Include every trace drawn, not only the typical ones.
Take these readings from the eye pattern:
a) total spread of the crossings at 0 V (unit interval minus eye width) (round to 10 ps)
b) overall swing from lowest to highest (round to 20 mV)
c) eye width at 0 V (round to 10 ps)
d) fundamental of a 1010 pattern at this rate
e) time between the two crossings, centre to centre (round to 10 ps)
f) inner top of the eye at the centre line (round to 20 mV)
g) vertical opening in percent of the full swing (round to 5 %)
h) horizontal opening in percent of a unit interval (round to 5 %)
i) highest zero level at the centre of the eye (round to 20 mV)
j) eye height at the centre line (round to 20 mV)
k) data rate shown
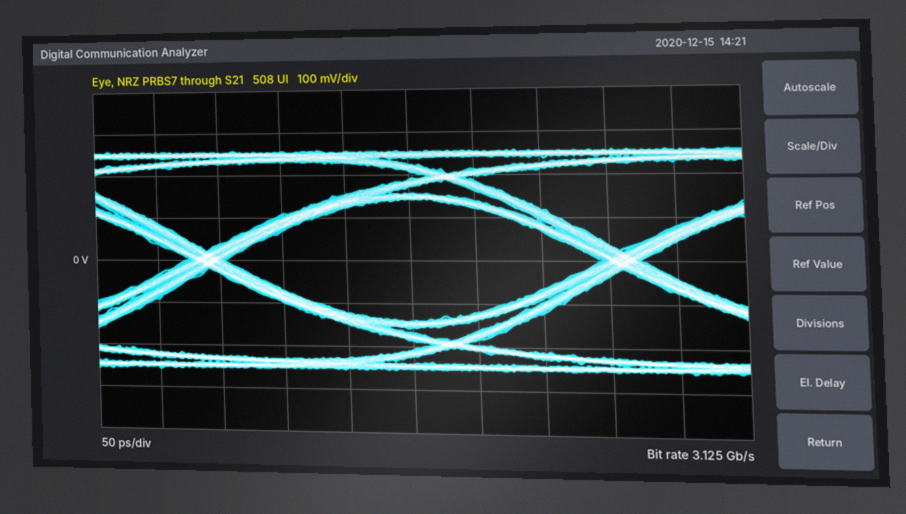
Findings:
30 ps
520 mV
290 ps
1.5625 GHz
320 ps
140 mV
55 %
90 %
-140 mV
280 mV
3.125 Gb/s
